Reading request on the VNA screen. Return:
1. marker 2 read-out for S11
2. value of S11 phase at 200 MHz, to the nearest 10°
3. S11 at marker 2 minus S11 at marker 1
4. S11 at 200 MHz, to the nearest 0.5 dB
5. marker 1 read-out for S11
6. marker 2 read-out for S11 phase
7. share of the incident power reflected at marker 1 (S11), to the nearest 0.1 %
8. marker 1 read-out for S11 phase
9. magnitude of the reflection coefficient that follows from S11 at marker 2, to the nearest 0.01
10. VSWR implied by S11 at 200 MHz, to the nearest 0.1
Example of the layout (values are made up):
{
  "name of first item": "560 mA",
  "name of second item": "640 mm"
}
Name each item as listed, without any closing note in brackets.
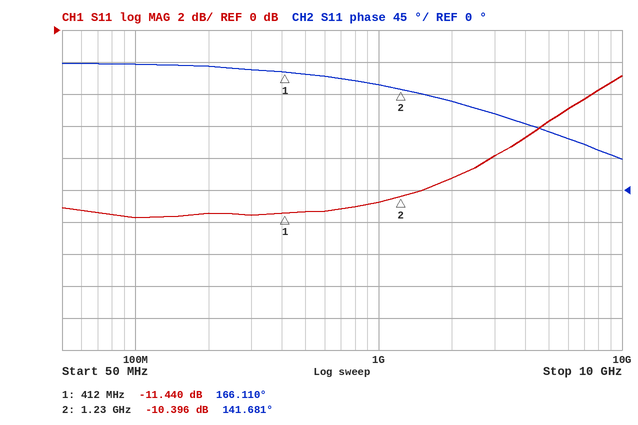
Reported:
{
  "marker 2 read-out for S11": "-10.396 dB",
  "value of S11 phase at 200 MHz, to the nearest 10°": "170°",
  "S11 at marker 2 minus S11 at marker 1": "1.044 dB",
  "S11 at 200 MHz, to the nearest 0.5 dB": "-11.5 dB",
  "marker 1 read-out for S11": "-11.440 dB",
  "marker 2 read-out for S11 phase": "141.681°",
  "share of the incident power reflected at marker 1 (S11), to the nearest 0.1 %": "7.2 %",
  "marker 1 read-out for S11 phase": "166.110°",
  "magnitude of the reflection coefficient that follows from S11 at marker 2, to the nearest 0.01": "0.30",
  "VSWR implied by S11 at 200 MHz, to the nearest 0.1": "1.7"
}
